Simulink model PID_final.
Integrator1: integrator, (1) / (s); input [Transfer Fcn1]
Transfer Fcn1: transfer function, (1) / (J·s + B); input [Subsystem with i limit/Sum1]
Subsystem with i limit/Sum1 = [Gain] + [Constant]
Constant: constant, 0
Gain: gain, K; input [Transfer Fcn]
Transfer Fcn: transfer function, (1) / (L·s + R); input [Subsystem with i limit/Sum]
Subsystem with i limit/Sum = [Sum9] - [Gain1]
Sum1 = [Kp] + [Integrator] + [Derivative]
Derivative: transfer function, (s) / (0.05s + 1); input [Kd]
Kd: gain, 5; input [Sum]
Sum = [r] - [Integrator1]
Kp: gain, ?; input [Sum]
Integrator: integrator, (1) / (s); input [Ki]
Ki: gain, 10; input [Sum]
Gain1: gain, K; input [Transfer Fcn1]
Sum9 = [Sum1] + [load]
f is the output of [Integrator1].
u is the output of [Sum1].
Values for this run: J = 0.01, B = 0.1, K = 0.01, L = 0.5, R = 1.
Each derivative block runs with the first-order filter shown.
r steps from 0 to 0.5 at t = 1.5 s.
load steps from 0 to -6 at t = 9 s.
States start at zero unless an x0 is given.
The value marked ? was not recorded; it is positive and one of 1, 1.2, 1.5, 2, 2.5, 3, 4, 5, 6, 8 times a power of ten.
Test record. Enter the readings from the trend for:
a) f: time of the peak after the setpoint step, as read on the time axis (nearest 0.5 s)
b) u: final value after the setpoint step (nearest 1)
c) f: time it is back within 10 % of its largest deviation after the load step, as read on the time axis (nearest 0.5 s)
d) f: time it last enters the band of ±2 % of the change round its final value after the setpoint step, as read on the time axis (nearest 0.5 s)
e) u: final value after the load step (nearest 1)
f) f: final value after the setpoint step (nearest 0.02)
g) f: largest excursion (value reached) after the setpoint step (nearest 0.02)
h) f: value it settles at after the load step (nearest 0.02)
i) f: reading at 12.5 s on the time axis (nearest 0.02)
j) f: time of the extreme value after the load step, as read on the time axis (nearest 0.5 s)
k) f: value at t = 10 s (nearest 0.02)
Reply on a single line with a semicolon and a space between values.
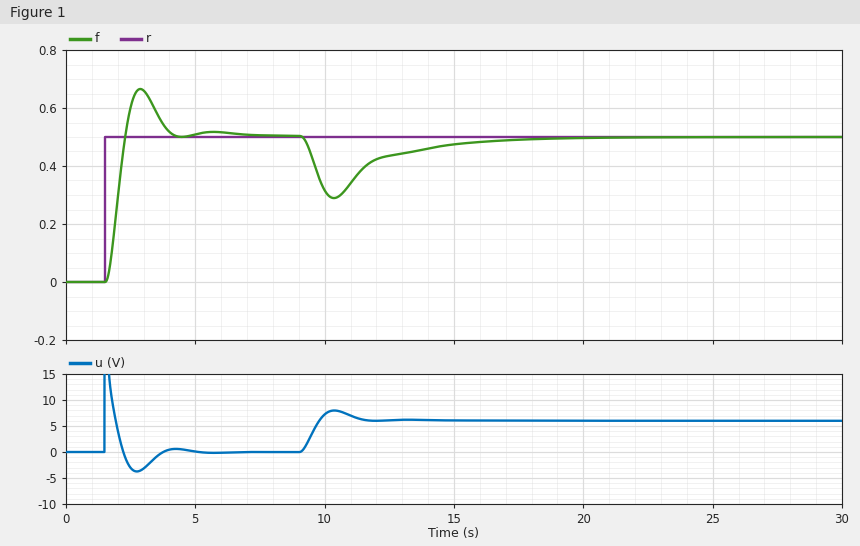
3.0 s; 0; 15.5 s; 6.5 s; 6; 0.50; 0.66; 0.50; 0.44; 10.5 s; 0.32
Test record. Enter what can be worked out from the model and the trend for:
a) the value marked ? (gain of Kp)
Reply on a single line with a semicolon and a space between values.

30
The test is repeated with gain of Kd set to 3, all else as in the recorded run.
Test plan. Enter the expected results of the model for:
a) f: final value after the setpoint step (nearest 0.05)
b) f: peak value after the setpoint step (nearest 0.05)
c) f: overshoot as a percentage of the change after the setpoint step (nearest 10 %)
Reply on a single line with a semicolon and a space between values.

0.50; 0.70; 40 %
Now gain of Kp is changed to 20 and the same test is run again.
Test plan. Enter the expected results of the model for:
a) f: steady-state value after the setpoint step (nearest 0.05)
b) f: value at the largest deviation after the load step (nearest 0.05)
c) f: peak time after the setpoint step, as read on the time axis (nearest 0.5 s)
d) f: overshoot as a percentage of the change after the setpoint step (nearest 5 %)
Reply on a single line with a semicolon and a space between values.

0.50; 0.25; 3.5 s; 30 %
